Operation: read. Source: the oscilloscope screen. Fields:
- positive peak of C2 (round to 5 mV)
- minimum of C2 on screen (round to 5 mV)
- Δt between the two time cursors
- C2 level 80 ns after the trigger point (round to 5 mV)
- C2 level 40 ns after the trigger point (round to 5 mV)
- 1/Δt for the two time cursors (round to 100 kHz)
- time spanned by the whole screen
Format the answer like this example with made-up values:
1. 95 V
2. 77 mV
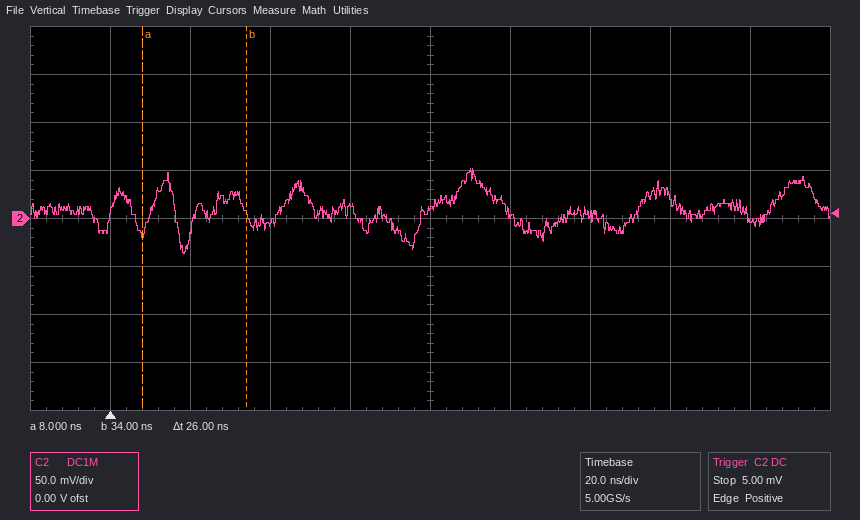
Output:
1. 50 mV
2. -35 mV
3. 26 ns
4. 10 mV
5. -5 mV
6. 38.5 MHz
7. 200 ns
